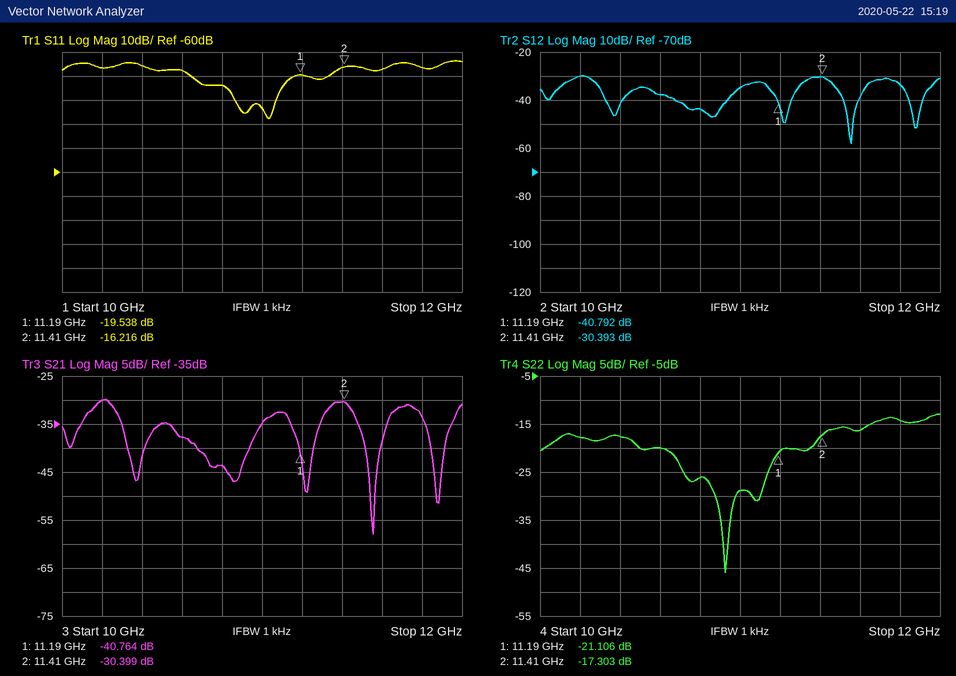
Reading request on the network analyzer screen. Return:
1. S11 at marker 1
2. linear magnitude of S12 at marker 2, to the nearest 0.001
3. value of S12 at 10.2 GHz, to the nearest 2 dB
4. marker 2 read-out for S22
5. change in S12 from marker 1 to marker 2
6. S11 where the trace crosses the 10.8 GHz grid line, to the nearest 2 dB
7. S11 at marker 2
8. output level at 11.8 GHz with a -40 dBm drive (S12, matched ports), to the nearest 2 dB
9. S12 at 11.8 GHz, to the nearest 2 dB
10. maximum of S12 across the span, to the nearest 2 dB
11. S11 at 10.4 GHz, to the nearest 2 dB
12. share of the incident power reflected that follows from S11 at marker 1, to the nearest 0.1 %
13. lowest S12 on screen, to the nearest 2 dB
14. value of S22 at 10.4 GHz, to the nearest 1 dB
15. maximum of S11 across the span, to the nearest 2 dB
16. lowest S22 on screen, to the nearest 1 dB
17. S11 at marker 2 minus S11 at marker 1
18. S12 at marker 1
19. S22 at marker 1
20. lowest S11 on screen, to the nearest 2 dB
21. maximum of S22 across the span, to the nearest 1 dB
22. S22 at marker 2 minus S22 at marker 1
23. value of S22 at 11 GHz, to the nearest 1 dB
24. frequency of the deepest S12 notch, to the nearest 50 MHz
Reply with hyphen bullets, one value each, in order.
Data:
- -19.538 dB
- 0.030
- -30 dB
- -17.303 dB
- 10.399 dB
- -24 dB
- -16.216 dB
- -74 dBm
- -34 dB
- -30 dB
- -16 dB
- 1.1 %
- -58 dB
- -18 dB
- -14 dB
- -46 dB
- 3.322 dB
- -40.792 dB
- -21.106 dB
- -38 dB
- -13 dB
- 3.803 dB
- -29 dB
- 11.55 GHz
